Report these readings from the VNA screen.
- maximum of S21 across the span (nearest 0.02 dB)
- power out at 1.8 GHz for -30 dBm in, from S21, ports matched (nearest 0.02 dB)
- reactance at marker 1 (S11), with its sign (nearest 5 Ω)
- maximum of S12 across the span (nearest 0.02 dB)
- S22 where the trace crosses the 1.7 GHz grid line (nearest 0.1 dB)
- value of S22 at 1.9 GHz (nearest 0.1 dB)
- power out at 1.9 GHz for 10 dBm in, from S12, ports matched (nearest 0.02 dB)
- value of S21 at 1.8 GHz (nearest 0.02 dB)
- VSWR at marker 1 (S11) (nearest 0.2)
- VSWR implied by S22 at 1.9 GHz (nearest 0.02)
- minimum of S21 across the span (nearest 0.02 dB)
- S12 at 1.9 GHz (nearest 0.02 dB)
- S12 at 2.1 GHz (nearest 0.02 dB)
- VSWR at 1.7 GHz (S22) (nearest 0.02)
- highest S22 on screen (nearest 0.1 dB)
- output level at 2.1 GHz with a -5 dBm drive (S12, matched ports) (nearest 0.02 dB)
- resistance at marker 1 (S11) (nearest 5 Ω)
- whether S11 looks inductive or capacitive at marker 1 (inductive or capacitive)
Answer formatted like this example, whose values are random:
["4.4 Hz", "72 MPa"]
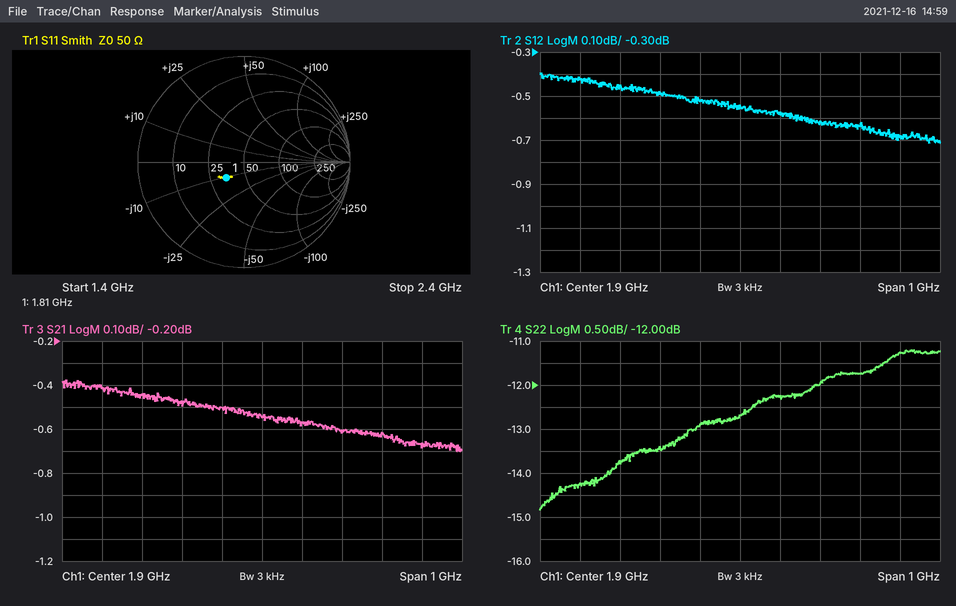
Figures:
["-0.38 dB", "-30.50 dBm", "-10 Ω", "-0.40 dB", "-13.4 dB", "-12.7 dB", "9.46 dBm", "-0.50 dB", "1.6", "1.60", "-0.70 dB", "-0.54 dB", "-0.62 dB", "1.54", "-11.2 dB", "-5.62 dBm", "35 Ω", "capacitive"]
